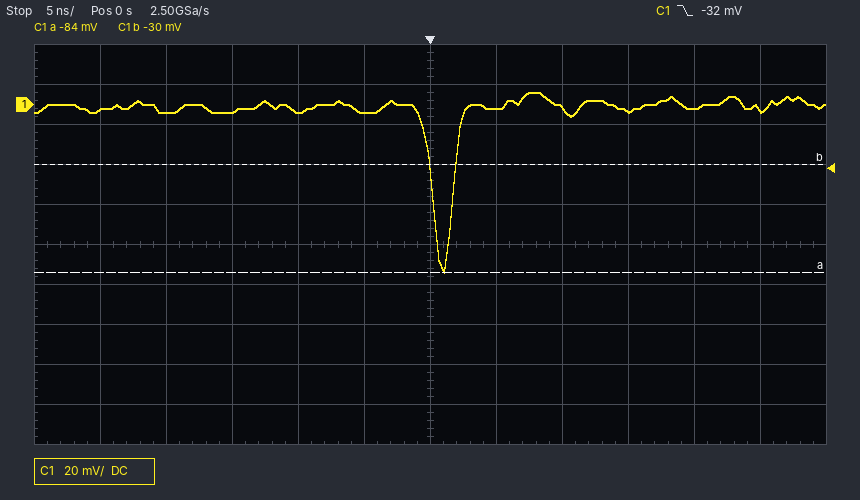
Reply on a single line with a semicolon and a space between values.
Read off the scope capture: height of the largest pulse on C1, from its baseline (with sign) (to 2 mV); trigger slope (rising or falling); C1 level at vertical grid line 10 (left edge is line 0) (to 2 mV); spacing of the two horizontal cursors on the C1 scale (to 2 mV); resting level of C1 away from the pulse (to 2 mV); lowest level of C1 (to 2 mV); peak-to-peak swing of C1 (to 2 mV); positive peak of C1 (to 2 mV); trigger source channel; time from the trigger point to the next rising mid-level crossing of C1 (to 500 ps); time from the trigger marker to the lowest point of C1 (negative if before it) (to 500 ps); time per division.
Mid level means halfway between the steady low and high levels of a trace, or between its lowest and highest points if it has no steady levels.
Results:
-84 mV; falling; -2 mV; 54 mV; 0 mV; -84 mV; 90 mV; 6 mV; C1; 2.0 ns; +1.0 ns; 5 ns
